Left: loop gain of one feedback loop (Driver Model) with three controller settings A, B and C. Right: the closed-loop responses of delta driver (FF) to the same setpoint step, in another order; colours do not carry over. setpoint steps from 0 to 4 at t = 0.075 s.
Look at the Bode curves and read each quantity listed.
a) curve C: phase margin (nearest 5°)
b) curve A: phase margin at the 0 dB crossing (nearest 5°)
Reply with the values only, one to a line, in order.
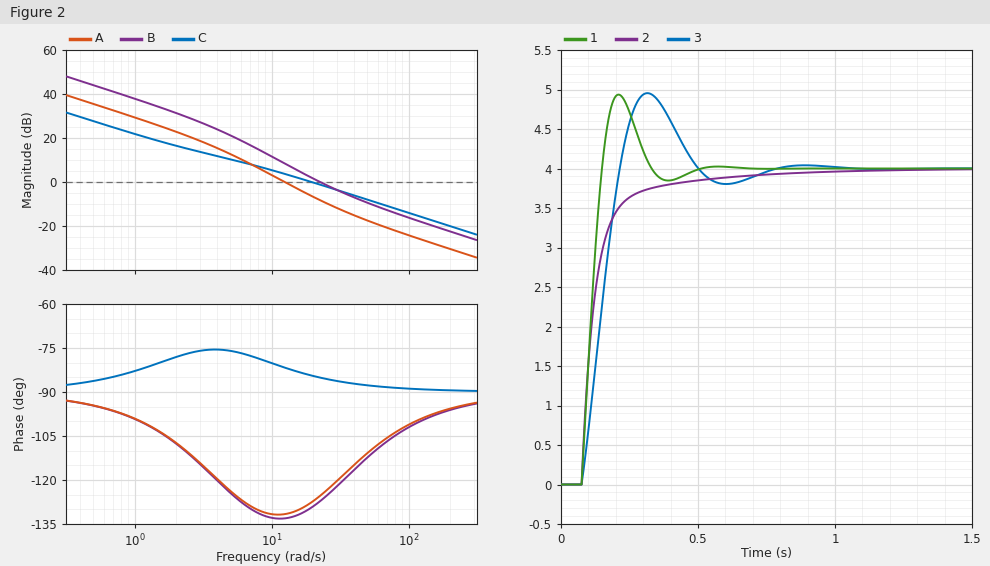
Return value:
95°
50°
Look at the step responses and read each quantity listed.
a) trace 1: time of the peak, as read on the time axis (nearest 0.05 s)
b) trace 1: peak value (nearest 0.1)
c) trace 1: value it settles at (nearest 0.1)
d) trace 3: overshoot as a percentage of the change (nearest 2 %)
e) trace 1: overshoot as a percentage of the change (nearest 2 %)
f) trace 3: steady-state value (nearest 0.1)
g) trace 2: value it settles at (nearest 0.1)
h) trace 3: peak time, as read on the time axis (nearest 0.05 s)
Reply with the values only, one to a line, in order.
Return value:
0.20 s
4.9
4.0
24 %
24 %
4.0
4.0
0.30 s
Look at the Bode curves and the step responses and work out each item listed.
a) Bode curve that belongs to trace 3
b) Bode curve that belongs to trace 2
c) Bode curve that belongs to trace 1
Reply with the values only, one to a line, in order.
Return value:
A
C
B
